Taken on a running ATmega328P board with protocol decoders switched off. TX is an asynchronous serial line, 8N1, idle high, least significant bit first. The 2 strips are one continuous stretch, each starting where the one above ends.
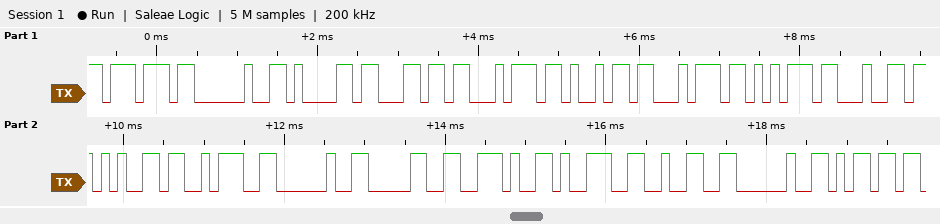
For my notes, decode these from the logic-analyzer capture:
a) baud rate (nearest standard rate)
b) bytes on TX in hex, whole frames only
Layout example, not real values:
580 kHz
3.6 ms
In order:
9600 baud
0x77 0x20 0x61 0x6C 0x74 0x69 0x74 0x75 0x64 0x65 0x3A 0x20 0x30 0x2E 0x39 0x32 0x20 0x6D
